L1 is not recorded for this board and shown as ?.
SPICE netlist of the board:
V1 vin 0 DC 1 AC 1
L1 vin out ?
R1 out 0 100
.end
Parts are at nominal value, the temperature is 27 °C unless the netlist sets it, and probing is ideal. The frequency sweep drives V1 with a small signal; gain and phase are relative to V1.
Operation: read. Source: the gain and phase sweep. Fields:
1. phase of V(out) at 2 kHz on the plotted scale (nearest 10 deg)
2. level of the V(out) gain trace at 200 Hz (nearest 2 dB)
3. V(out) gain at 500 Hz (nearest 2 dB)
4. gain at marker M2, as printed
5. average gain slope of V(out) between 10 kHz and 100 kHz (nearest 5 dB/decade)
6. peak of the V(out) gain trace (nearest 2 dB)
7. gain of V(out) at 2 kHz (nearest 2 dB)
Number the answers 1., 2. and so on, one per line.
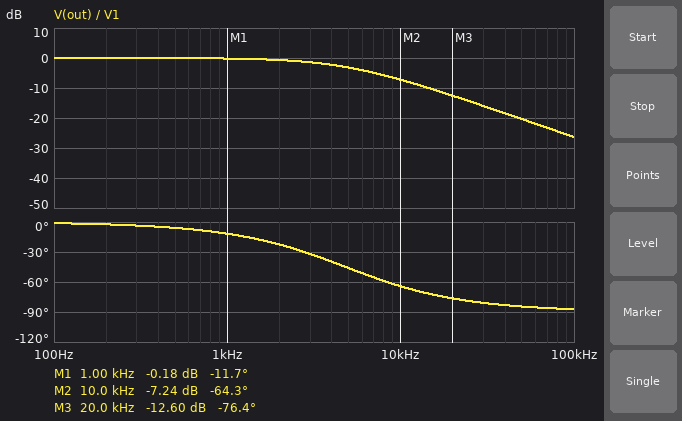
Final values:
1. -20 deg
2. 0 dB
3. 0 dB
4. -7.24 dB
5. -20 dB/decade
6. 0 dB
7. 0 dB
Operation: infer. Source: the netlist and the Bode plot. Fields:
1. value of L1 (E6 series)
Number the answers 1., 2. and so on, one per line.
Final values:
1. 3.3 mH
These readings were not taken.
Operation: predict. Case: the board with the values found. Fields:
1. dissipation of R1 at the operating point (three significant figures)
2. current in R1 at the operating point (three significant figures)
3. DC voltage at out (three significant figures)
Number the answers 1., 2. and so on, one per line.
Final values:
1. 10.0 mW
2. 10.0 mA
3. 1.00 V
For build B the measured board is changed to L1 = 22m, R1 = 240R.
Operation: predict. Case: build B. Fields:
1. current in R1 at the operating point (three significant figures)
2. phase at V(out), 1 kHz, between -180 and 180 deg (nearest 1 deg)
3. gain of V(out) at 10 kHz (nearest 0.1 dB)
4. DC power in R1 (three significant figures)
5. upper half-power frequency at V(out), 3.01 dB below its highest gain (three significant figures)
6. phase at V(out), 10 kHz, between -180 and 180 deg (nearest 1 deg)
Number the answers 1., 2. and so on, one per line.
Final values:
1. 4.17 mA
2. -30 deg
3. -15.3 dB
4. 4.17 mW
5. 1.74 kHz
6. -80 deg
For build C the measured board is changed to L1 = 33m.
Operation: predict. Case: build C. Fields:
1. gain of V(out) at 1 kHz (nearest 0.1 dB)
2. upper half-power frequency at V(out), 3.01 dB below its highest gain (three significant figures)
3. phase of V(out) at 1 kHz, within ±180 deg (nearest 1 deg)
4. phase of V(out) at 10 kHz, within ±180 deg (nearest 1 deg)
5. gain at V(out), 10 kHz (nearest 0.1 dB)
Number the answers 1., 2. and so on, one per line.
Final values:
1. -7.2 dB
2. 482 Hz
3. -64 deg
4. -87 deg
5. -26.3 dB
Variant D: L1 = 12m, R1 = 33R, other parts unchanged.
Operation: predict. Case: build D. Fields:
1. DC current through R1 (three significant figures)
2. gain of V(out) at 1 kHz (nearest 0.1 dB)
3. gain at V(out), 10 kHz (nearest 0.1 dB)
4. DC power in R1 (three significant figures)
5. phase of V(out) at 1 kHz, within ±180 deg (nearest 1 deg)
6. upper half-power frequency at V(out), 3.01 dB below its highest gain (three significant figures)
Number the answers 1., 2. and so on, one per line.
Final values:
1. 30.3 mA
2. -7.9 dB
3. -27.2 dB
4. 30.3 mW
5. -66 deg
6. 438 Hz
